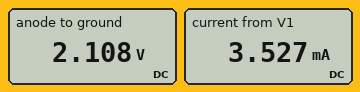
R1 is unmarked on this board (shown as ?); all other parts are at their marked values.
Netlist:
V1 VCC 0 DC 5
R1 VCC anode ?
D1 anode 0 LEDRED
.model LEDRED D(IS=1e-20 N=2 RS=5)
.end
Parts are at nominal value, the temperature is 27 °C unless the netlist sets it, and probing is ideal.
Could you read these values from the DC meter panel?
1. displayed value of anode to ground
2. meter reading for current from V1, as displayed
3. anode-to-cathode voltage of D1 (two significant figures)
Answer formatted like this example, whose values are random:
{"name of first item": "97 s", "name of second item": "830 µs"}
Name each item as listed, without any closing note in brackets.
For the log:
{"displayed value of anode to ground": "2.108 V", "meter reading for current from V1, as displayed": "3.527 mA", "anode-to-cathode voltage of D1": "2.1 V"}
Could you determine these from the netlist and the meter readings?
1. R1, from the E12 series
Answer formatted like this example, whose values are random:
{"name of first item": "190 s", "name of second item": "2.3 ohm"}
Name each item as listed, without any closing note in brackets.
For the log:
{"R1, from the E12 series": "820 Ω"}
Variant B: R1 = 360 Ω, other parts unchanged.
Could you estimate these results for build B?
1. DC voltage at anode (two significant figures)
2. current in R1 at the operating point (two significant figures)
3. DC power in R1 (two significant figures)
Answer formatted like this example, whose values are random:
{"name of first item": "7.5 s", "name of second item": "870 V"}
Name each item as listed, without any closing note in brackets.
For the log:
{"DC voltage at anode": "2.2 V", "current in R1 at the operating point": "7.9 mA", "DC power in R1": "22 mW"}
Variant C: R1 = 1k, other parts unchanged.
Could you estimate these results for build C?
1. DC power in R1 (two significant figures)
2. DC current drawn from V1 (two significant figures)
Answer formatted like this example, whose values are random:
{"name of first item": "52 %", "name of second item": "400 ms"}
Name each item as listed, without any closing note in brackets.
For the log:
{"DC power in R1": "8.4 mW", "DC current drawn from V1": "2.9 mA"}
